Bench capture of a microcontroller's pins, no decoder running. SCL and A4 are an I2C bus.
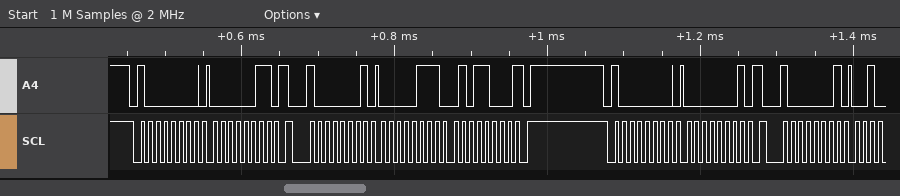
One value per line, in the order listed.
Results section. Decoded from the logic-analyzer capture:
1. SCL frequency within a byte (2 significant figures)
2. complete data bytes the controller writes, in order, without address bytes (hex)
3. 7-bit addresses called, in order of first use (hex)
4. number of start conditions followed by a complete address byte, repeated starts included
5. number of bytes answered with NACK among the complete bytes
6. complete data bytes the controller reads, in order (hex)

100 kHz
03 01
0x40
4
1
07 58
